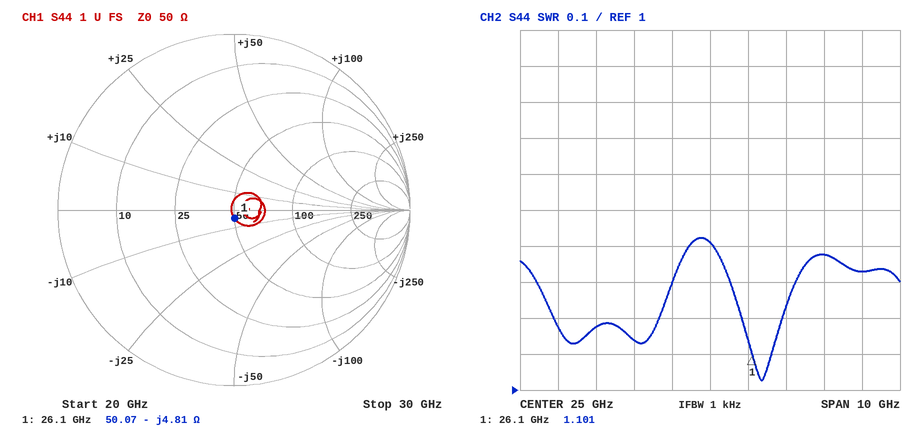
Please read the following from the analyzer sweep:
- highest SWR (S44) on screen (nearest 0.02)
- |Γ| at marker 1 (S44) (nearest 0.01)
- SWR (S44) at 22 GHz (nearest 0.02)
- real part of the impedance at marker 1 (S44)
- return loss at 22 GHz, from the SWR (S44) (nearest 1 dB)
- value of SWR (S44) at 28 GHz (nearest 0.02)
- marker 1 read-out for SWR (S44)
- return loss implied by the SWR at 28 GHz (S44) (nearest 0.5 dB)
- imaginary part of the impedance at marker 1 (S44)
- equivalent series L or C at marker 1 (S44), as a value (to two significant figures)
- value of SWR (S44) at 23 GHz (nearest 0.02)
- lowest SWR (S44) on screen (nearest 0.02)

1.42
0.05
1.18
50.07 Ω
22 dB
1.38
1.101
16.0 dB
-4.81 Ω
1.3 pF
1.14
1.02
